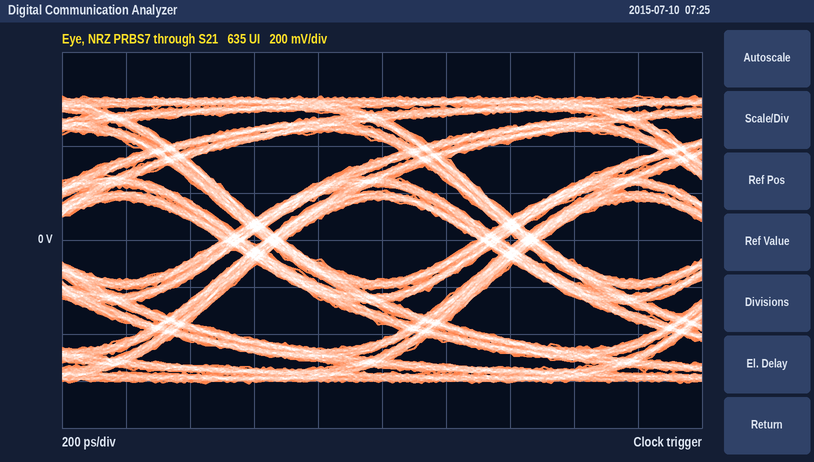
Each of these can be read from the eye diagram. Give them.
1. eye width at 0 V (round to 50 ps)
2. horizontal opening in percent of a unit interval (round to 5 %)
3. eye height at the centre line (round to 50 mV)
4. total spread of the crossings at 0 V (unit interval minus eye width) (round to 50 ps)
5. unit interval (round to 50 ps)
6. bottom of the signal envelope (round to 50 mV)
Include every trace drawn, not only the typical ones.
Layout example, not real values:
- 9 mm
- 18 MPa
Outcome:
- 600 ps
- 75 %
- 350 mV
- 200 ps
- 800 ps
- -600 mV
